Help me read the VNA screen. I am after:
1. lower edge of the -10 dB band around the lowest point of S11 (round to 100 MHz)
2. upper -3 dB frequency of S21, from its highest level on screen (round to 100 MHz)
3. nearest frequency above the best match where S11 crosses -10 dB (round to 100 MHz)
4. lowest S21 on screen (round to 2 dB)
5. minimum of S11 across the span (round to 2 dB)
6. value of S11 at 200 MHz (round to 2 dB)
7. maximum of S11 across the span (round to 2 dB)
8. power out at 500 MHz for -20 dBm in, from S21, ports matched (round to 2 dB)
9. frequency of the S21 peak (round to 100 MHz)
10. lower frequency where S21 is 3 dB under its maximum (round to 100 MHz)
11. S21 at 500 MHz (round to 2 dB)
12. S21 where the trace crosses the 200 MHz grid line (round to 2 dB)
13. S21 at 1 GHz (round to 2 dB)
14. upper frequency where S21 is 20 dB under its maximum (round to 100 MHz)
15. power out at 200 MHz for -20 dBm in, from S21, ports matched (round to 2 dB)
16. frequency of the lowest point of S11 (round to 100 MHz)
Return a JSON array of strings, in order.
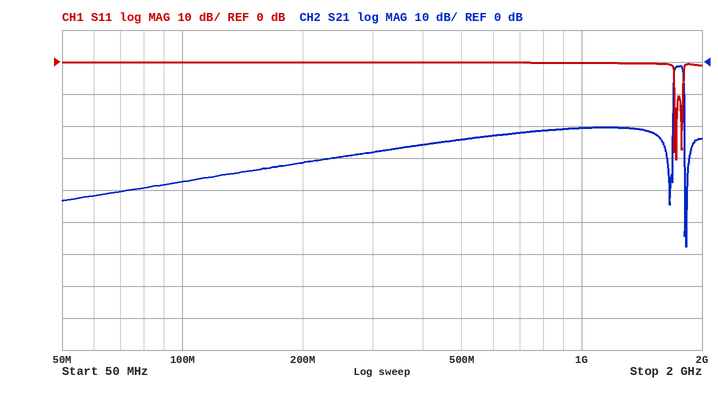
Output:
["1.7 GHz", "1.8 GHz", "1.8 GHz", "-58 dB", "-30 dB", "0 dB", "0 dB", "-44 dBm", "1.8 GHz", "1.7 GHz", "-24 dB", "-32 dB", "-20 dB", "1.8 GHz", "-52 dBm", "1.7 GHz"]
